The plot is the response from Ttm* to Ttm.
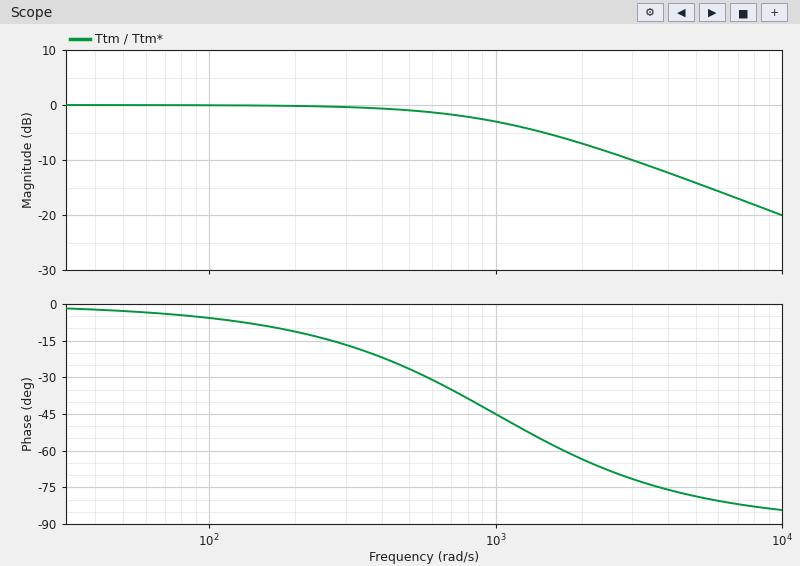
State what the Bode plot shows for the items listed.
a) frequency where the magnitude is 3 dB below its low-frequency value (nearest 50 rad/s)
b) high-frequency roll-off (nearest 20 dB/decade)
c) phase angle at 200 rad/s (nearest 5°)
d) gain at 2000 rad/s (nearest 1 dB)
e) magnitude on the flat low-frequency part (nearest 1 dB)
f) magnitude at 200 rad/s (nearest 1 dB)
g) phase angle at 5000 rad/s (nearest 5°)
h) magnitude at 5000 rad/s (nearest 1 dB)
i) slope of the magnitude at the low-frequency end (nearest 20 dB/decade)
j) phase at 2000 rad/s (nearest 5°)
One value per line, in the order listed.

1000 rad/s
-20 dB/decade
-10°
-7 dB
0 dB
0 dB
-80°
-14 dB
0 dB/decade
-65°
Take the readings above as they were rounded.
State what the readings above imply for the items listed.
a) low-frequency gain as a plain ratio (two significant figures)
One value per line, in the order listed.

1.0
